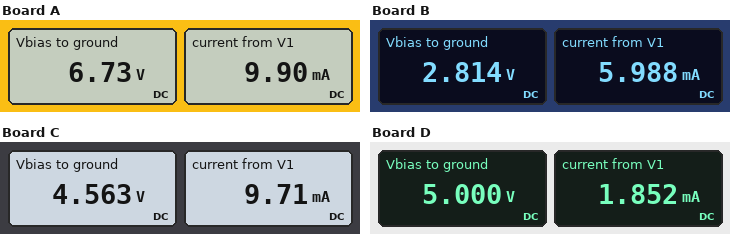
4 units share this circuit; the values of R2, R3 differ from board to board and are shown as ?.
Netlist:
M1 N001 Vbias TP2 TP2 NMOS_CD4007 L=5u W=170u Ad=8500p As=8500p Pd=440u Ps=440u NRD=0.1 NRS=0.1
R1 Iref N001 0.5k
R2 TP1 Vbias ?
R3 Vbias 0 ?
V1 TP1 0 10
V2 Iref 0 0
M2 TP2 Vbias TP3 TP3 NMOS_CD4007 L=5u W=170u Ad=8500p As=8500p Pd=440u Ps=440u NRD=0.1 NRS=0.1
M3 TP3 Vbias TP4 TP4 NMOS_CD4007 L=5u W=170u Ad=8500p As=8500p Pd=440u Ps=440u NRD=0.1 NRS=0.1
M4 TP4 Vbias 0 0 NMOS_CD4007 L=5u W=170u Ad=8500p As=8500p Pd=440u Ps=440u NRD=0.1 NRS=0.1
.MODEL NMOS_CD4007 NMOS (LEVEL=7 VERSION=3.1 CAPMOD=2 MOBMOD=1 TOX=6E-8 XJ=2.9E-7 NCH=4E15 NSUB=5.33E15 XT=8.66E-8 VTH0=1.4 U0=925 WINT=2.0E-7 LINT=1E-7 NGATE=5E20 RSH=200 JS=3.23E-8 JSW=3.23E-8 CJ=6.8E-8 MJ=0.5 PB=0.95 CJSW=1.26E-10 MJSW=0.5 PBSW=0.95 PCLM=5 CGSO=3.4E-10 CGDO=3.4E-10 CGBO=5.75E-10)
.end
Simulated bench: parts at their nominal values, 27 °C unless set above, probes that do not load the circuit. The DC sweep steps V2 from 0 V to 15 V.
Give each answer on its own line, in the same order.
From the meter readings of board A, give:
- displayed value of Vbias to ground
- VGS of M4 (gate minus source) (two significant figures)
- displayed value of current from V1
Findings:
6.73 V
6.7 V
9.90 mA
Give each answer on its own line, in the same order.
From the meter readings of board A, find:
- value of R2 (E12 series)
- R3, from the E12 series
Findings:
330 Ω
680 Ω
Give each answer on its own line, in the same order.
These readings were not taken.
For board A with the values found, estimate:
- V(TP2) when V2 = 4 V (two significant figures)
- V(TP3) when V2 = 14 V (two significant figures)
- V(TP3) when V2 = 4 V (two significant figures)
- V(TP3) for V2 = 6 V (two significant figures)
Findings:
1.8 V
1.6 V
1.1 V
1.5 V
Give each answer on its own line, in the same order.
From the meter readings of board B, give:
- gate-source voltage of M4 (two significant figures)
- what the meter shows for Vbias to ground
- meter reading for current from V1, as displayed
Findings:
2.8 V
2.814 V
5.988 mA
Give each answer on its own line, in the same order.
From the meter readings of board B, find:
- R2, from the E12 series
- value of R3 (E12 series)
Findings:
1.2 kΩ
470 Ω
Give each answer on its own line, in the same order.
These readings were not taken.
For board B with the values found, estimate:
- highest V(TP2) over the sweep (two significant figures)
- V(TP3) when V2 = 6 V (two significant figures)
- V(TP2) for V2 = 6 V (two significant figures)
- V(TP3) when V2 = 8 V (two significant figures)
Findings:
770 mV
410 mV
710 mV
420 mV
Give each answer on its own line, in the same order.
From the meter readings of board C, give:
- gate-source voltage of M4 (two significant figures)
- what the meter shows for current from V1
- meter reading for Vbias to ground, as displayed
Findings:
4.6 V
9.71 mA
4.563 V
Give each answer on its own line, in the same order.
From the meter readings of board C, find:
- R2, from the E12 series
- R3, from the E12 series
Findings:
560 Ω
470 Ω
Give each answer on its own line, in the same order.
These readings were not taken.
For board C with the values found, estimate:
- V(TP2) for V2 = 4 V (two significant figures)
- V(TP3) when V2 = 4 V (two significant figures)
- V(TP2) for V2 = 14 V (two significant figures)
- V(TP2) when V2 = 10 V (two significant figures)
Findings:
1.5 V
890 mV
1.6 V
1.6 V
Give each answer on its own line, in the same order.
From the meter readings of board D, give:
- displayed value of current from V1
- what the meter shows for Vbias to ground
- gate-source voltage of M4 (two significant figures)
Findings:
1.852 mA
5.000 V
5.0 V
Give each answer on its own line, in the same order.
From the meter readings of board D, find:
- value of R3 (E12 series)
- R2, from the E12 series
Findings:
2.7 kΩ
2.7 kΩ
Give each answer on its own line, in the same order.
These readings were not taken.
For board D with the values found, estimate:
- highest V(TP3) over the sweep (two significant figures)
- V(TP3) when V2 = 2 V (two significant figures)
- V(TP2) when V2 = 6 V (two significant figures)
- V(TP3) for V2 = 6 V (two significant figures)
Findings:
1.1 V
620 mV
1.7 V
1.0 V
